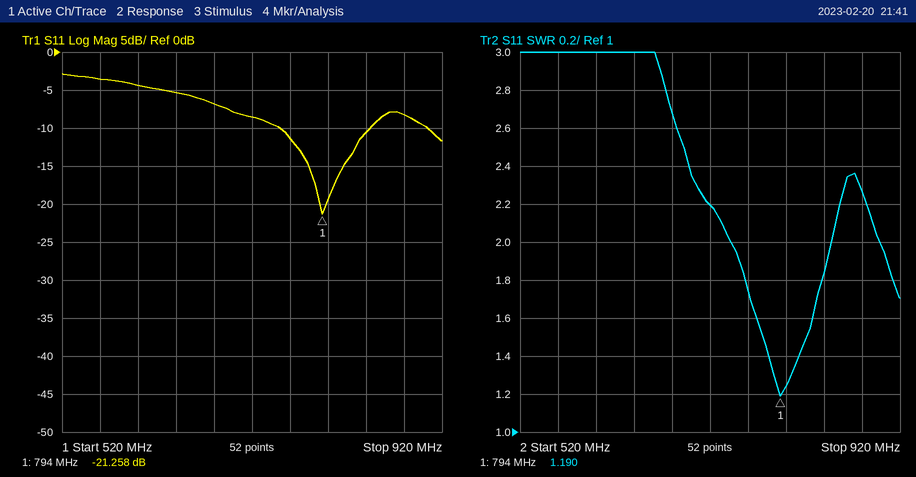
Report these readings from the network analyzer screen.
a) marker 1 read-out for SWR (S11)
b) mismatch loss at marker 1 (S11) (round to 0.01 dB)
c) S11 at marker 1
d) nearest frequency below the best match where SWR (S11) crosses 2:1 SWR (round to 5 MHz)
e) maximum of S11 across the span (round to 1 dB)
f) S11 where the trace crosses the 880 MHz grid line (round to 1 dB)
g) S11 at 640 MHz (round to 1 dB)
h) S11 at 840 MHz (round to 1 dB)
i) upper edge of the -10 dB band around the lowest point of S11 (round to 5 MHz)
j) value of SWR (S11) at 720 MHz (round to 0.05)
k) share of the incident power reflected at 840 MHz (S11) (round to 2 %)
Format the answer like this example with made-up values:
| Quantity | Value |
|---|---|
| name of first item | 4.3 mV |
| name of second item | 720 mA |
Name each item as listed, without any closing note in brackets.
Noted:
| Quantity | Value |
|---|---|
| marker 1 read-out for SWR | 1.190 |
| mismatch loss at marker 1 (S11) | 0.03 dB |
| S11 at marker 1 | -21.258 dB |
| nearest frequency below the best match where SWR (S11) crosses 2:1 SWR | 740 MHz |
| maximum of S11 across the span | -3 dB |
| S11 where the trace crosses the 880 MHz grid line | -8 dB |
| S11 at 640 MHz | -5 dB |
| S11 at 840 MHz | -11 dB |
| upper edge of the -10 dB band around the lowest point of S11 | 845 MHz |
| value of SWR (S11) at 720 MHz | 2.20 |
| share of the incident power reflected at 840 MHz (S11) | 8 % |
